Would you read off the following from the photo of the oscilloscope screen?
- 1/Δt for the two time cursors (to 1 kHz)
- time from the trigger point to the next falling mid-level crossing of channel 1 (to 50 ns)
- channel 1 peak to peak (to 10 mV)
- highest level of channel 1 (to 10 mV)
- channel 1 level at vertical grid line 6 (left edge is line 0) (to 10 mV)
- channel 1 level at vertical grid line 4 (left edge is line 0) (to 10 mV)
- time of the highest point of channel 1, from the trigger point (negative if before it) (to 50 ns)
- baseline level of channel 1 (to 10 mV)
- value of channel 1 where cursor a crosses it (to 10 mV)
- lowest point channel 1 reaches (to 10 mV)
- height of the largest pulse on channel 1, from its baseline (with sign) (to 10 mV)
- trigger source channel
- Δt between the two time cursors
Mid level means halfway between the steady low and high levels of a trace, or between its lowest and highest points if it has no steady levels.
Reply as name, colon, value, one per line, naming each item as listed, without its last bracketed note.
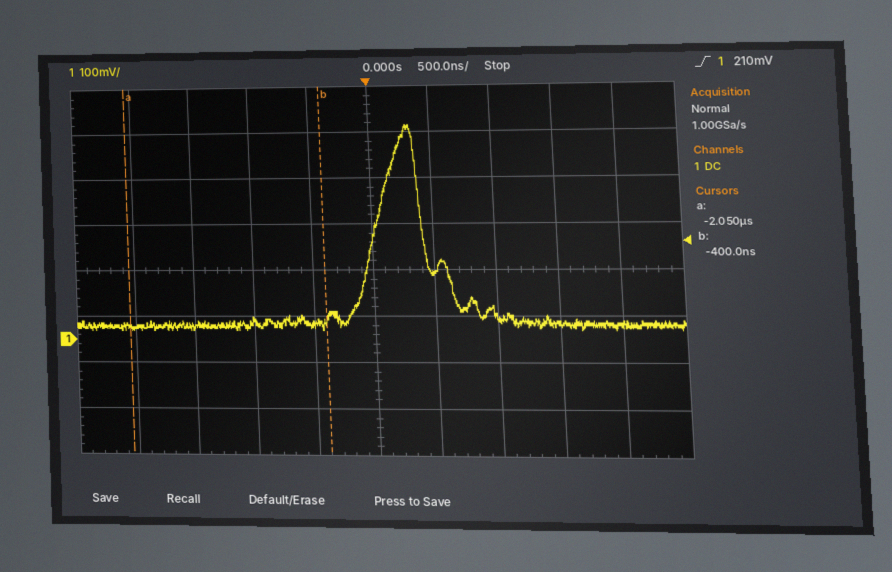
1/Δt for the two time cursors: 606 kHz
time from the trigger point to the next falling mid-level crossing of channel 1: 400 ns
channel 1 peak to peak: 440 mV
highest level of channel 1: 460 mV
channel 1 level at vertical grid line 6 (left edge is line 0): 140 mV
channel 1 level at vertical grid line 4 (left edge is line 0): 30 mV
time of the highest point of channel 1, from the trigger point (negative if before it): +300 ns
baseline level of channel 1: 30 mV
value of channel 1 where cursor a crosses it: 30 mV
lowest point channel 1 reaches: 20 mV
height of the largest pulse on channel 1, from its baseline (with sign): +430 mV
trigger source channel: channel 1
Δt between the two time cursors: 1.65 µs
